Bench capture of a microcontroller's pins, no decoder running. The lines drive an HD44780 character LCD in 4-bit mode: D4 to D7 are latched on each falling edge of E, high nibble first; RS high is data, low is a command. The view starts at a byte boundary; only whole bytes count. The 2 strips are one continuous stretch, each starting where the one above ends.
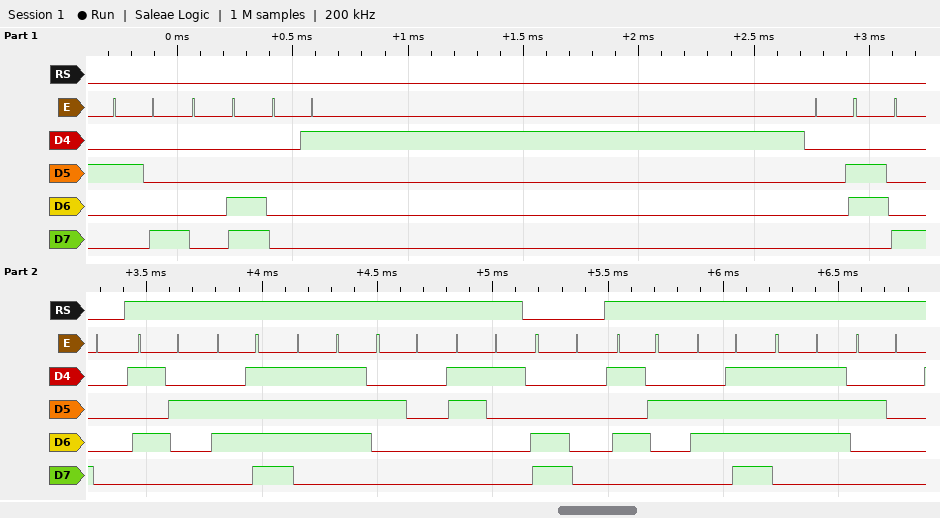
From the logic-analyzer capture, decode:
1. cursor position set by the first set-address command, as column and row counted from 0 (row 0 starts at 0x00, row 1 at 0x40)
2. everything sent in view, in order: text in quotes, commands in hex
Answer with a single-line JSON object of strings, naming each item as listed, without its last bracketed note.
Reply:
{"cursor position set by the first set-address command, as column and row counted from 0": "column 0, row 0", "everything sent in view, in order: text in quotes, commands in hex": "0x28 0x0C 0x01 0x06 0x80 \"Row 1\" 0xC0 \"Row \""}
